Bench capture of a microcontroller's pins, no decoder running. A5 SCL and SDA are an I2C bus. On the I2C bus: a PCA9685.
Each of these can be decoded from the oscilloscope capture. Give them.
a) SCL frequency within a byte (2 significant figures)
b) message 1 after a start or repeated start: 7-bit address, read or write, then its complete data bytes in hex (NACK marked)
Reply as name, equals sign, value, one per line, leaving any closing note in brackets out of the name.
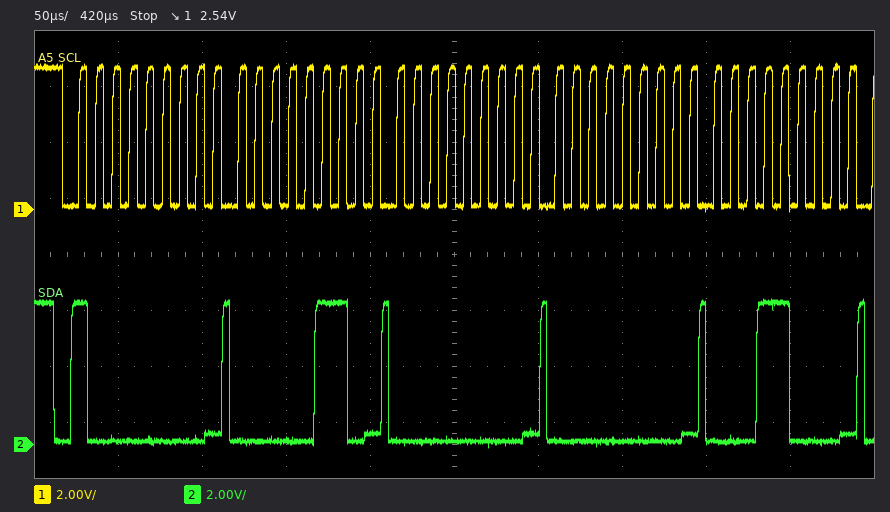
SCL frequency within a byte = 100 kHz
message 1 after a start or repeated start: 7-bit address, read or write, then its complete data bytes in hex = 0x40 write: 06 00 00 18
